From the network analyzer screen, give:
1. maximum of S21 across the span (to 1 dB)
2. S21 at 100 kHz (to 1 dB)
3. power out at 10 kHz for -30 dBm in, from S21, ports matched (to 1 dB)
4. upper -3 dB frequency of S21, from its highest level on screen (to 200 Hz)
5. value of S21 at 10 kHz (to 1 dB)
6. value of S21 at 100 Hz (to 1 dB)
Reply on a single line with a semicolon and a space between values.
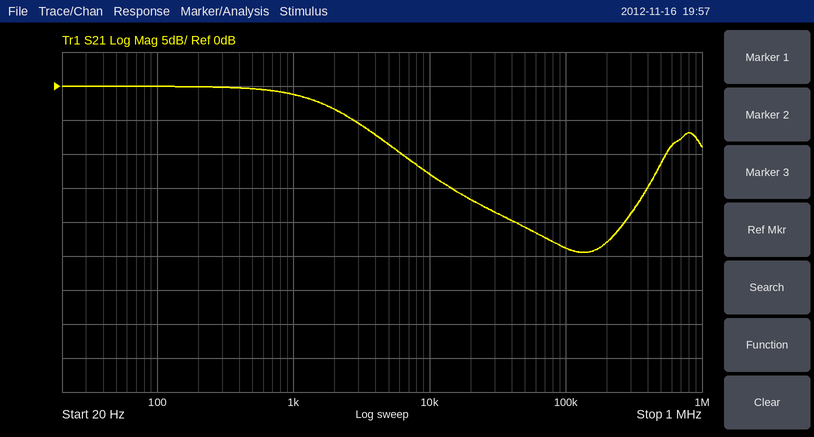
0 dB; -24 dB; -43 dBm; 1.8 kHz; -13 dB; 0 dB
